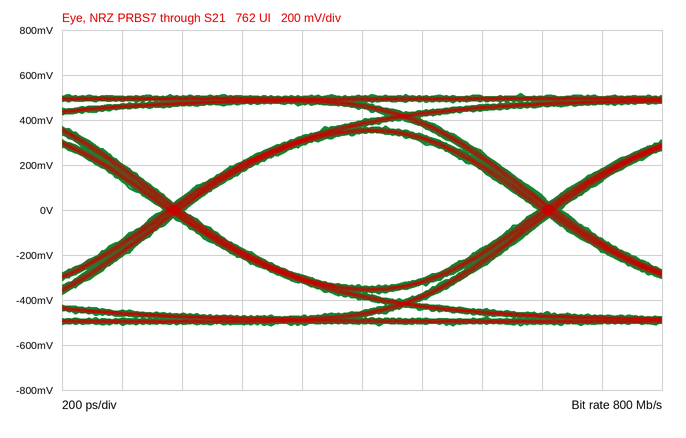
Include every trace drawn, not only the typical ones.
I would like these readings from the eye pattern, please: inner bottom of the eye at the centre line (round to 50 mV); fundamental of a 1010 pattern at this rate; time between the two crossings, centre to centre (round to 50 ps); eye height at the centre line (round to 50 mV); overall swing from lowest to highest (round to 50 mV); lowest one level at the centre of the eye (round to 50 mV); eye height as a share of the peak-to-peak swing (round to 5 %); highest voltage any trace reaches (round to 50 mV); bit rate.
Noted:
-350 mV
400 MHz
1.25 ns
700 mV
1.05 V
350 mV
65 %
500 mV
800 Mb/s
